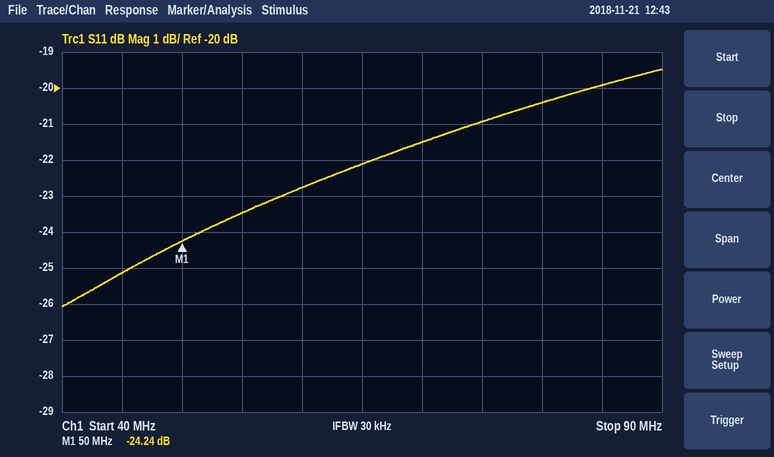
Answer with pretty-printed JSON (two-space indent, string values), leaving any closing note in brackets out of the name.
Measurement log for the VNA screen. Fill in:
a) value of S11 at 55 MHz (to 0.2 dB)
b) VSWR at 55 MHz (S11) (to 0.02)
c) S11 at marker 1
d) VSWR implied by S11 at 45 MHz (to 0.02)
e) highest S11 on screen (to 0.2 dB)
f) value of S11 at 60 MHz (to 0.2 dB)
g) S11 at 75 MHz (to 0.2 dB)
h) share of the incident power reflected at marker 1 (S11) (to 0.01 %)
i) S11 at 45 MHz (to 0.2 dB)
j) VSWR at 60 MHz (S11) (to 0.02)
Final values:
{
  "value of S11 at 55 MHz": "-23.4 dB",
  "VSWR at 55 MHz (S11)": "1.14",
  "S11 at marker 1": "-24.24 dB",
  "VSWR implied by S11 at 45 MHz": "1.12",
  "highest S11 on screen": "-19.4 dB",
  "value of S11 at 60 MHz": "-22.8 dB",
  "S11 at 75 MHz": "-21.0 dB",
  "share of the incident power reflected at marker 1 (S11)": "0.38 %",
  "S11 at 45 MHz": "-25.2 dB",
  "VSWR at 60 MHz (S11)": "1.16"
}
